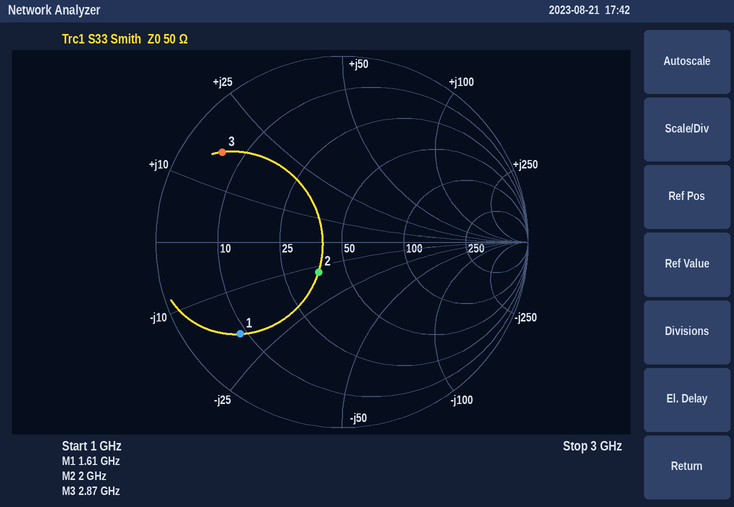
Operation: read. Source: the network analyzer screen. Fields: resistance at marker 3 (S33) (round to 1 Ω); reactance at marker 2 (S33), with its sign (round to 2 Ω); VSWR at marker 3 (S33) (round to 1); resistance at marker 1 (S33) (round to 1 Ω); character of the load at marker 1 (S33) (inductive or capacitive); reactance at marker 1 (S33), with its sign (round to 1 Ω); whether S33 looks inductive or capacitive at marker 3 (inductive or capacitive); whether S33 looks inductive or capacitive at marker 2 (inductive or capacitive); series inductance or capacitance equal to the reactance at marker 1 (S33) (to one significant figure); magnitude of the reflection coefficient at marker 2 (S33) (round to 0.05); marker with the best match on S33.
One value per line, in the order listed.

6 Ω
-12 Ω
9
9 Ω
capacitive
-19 Ω
inductive
capacitive
5 pF
0.20
marker 2
